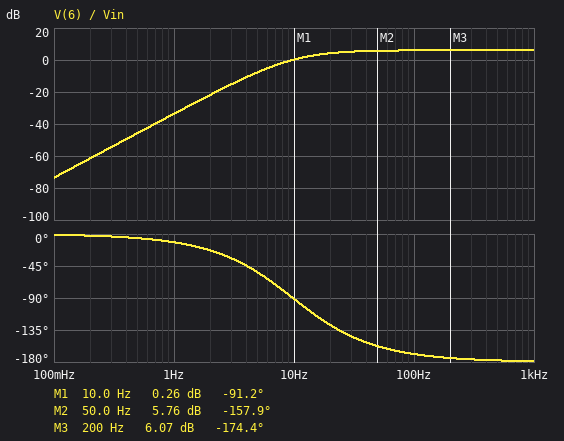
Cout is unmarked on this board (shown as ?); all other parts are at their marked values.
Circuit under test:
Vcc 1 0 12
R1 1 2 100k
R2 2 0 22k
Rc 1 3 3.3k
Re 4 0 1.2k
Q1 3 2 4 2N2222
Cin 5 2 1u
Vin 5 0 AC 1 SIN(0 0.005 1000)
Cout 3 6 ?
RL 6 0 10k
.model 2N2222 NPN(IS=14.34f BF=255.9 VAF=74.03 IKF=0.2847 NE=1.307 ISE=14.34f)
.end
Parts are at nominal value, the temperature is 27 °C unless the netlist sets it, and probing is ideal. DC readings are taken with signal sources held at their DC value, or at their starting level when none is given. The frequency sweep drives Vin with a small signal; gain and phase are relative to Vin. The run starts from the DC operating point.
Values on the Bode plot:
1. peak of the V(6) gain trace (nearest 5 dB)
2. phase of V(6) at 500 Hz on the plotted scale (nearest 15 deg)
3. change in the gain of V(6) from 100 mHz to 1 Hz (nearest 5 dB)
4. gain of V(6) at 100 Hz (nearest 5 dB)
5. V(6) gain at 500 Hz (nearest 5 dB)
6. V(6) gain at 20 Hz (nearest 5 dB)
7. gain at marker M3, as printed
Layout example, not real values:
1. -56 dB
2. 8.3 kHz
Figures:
1. 5 dB
2. -180 deg
3. 40 dB
4. 5 dB
5. 5 dB
6. 5 dB
7. 6.07 dB
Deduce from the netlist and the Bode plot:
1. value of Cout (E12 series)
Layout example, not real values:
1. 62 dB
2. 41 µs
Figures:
1. 1.2 µF
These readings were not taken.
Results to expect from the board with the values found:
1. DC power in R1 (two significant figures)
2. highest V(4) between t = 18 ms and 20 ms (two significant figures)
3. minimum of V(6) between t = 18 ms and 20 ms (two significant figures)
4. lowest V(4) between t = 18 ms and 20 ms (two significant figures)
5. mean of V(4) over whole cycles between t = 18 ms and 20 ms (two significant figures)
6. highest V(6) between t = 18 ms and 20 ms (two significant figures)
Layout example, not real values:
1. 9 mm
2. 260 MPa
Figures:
1. 990 µW
2. 1.4 V
3. -10 mV
4. 1.4 V
5. 1.4 V
6. 10 mV
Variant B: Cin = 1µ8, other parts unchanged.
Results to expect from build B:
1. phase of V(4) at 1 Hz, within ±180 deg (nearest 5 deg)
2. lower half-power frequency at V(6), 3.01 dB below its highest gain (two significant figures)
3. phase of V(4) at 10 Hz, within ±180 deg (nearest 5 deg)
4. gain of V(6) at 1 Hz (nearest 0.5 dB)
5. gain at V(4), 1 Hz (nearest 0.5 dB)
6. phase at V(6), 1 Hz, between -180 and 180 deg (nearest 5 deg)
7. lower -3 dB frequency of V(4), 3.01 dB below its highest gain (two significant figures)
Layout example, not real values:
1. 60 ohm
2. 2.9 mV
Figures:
1. 80 deg
2. 12 Hz
3. 30 deg
4. -28.5 dB
5. -15.0 dB
6. -15 deg
7. 5.3 Hz
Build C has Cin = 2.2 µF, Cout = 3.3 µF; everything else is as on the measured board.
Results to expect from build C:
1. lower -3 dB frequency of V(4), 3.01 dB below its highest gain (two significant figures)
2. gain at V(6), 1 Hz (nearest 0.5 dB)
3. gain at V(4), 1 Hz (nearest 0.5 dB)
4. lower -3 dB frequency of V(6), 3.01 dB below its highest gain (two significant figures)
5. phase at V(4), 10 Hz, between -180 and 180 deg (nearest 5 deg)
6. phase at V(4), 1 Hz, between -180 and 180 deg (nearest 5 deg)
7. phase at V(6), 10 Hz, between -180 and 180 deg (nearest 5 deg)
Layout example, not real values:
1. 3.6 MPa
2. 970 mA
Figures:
1. 4.4 Hz
2. -18.5 dB
3. -13.0 dB
4. 6.2 Hz
5. 25 deg
6. 75 deg
7. -135 deg
